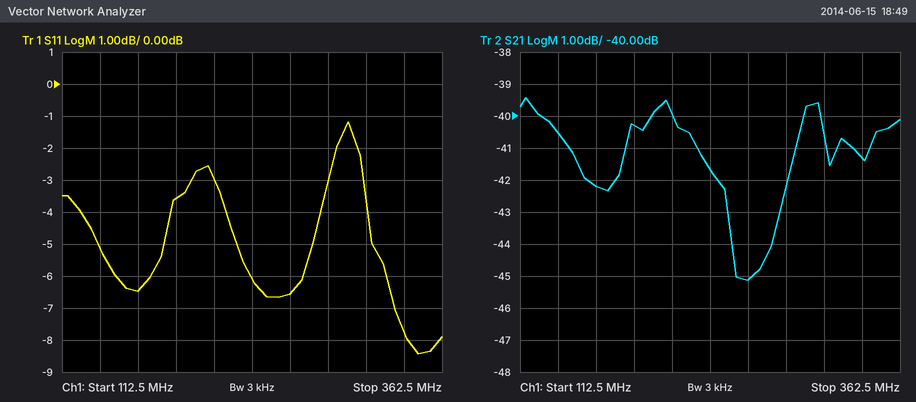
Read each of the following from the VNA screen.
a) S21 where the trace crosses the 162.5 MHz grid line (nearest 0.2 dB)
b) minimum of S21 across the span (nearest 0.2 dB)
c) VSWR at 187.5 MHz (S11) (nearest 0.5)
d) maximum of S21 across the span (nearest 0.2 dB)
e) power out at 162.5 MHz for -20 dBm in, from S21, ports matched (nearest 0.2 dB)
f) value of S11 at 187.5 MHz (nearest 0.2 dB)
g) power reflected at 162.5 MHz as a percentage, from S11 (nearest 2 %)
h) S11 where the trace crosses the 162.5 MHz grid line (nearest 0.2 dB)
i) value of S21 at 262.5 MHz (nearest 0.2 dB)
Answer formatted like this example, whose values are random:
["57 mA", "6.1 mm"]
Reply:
["-42.2 dB", "-45.2 dB", "5.0", "-39.4 dB", "-62.2 dBm", "-3.6 dB", "22 %", "-6.4 dB", "-45.2 dB"]
